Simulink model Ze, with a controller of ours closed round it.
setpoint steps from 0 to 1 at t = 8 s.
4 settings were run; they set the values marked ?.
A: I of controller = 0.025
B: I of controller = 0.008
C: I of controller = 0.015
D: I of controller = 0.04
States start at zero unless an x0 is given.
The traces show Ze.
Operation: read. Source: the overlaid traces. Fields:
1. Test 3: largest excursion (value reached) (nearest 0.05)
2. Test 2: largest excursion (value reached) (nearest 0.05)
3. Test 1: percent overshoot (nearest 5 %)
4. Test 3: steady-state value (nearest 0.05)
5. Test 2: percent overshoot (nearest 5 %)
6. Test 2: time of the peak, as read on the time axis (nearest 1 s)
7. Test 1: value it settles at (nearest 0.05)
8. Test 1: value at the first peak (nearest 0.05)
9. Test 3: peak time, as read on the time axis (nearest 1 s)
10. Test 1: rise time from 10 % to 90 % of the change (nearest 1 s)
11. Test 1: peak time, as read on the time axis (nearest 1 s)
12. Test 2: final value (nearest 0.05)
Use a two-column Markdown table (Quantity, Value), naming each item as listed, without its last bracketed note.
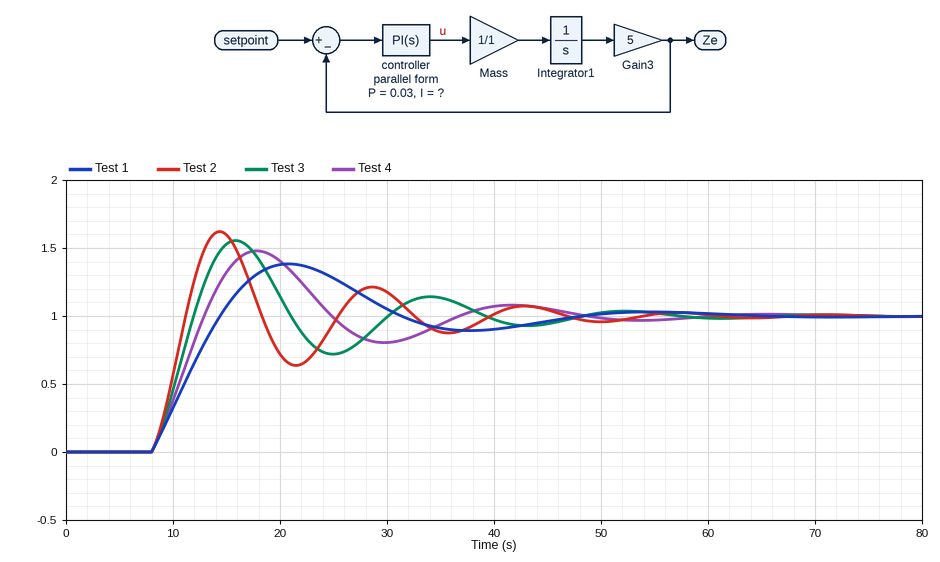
| Quantity | Value |
|---|---|
| Test 3: largest excursion (value reached) | 1.55 |
| Test 2: largest excursion (value reached) | 1.60 |
| Test 1: percent overshoot | 40 % |
| Test 3: steady-state value | 1.00 |
| Test 2: percent overshoot | 60 % |
| Test 2: time of the peak, as read on the time axis | 14 s |
| Test 1: value it settles at | 1.00 |
| Test 1: value at the first peak | 1.40 |
| Test 3: peak time, as read on the time axis | 16 s |
| Test 1: rise time from 10 % to 90 % of the change | 5 s |
| Test 1: peak time, as read on the time axis | 21 s |
| Test 2: final value | 1.00 |
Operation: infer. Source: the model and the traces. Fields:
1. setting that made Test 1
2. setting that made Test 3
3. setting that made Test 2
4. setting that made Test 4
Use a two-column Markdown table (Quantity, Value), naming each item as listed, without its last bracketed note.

| Quantity | Value |
|---|---|
| setting that made Test 1 | B |
| setting that made Test 3 | A |
| setting that made Test 2 | D |
| setting that made Test 4 | C |
